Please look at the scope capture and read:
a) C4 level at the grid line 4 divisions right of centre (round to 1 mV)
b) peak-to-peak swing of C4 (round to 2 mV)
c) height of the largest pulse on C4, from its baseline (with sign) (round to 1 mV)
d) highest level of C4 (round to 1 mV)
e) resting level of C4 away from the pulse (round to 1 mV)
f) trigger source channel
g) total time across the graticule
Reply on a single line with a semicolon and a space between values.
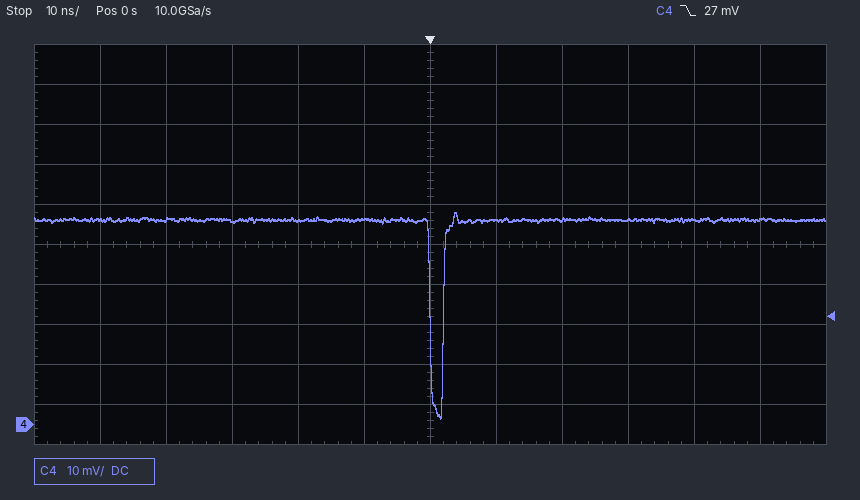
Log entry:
51 mV; 52 mV; -50 mV; 53 mV; 51 mV; C4; 120 ns
